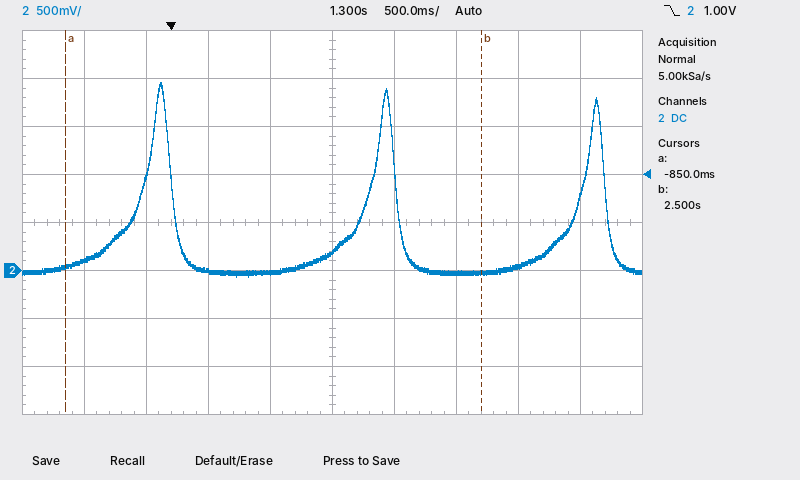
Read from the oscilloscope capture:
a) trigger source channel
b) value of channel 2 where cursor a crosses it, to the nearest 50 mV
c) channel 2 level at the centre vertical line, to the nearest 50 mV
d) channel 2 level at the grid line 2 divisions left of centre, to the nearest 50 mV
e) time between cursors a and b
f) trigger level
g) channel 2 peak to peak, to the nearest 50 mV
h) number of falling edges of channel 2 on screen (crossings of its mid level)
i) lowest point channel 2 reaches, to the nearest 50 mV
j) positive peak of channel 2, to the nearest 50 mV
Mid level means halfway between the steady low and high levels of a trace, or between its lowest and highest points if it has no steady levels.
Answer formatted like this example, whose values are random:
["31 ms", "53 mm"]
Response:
["channel 2", "50 mV", "200 mV", "0 mV", "3.35 s", "1.00 V", "2.00 V", "3", "-50 mV", "1.95 V"]
